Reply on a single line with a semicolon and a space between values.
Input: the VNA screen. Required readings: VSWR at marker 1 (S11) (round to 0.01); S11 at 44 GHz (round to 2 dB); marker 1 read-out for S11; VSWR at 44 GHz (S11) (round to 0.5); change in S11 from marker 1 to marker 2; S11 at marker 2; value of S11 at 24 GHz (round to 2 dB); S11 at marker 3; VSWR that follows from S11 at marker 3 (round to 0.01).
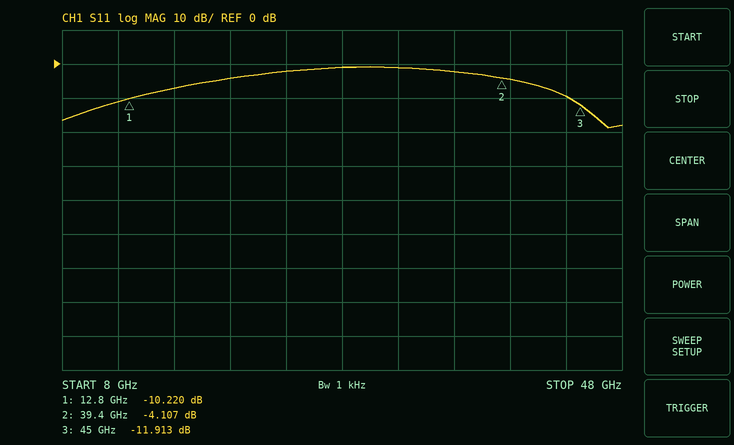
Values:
1.89; -10 dB; -10.220 dB; 2.0; 6.113 dB; -4.107 dB; -2 dB; -11.913 dB; 1.68
